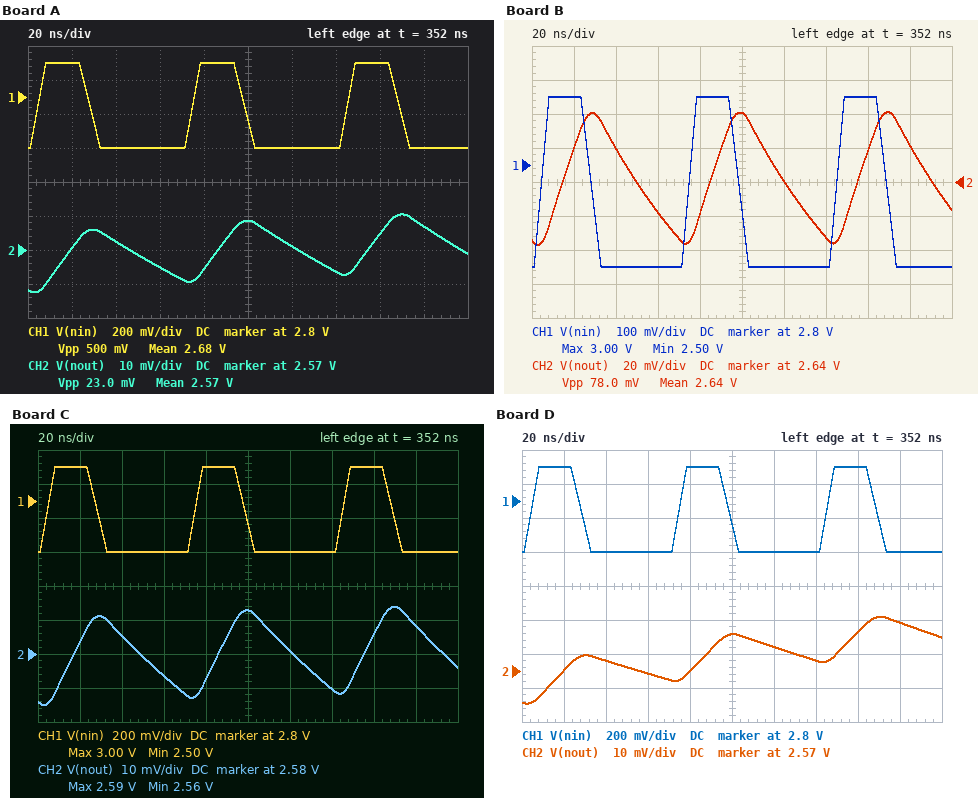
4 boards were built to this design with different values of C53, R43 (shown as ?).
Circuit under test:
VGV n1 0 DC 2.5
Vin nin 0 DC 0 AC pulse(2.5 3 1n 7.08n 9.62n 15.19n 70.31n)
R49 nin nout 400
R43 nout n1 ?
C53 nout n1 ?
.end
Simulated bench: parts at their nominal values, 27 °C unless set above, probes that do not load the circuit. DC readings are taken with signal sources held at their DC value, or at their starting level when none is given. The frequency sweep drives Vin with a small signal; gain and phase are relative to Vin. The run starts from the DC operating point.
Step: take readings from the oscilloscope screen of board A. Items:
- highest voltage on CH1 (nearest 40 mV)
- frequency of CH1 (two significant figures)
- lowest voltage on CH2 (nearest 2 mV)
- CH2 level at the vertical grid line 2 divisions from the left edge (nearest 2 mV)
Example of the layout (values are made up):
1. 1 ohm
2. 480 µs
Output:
1. 3.00 V
2. 14 MHz
3. 2.558 V
4. 2.572 V
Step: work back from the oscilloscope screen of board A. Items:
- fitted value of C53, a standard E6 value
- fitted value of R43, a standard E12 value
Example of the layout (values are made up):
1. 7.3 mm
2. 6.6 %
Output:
1. 1 nF
2. 330 Ω
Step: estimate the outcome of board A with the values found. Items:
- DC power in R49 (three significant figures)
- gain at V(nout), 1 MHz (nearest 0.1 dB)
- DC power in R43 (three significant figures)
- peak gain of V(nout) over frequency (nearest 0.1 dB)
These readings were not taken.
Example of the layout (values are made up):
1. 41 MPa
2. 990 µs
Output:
1. 4.69 mW
2. -10.5 dB
3. 3.87 mW
4. -6.9 dB
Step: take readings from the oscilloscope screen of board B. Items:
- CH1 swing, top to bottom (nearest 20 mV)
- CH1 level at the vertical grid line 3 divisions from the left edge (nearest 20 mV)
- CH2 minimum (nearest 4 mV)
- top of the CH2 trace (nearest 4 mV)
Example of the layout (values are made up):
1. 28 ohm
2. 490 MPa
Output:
1. 500 mV
2. 2.50 V
3. 2.604 V
4. 2.680 V
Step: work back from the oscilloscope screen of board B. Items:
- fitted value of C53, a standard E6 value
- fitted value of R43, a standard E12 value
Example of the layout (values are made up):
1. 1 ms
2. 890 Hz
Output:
1. 220 pF
2. 2.2 kΩ
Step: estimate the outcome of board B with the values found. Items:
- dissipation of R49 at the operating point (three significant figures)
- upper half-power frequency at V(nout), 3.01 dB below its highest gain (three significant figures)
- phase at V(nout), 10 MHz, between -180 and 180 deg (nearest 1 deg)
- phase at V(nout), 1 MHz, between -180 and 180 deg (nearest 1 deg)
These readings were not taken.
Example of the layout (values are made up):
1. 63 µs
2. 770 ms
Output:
1. 370 µW
2. 2.14 MHz
3. -78 deg
4. -25 deg
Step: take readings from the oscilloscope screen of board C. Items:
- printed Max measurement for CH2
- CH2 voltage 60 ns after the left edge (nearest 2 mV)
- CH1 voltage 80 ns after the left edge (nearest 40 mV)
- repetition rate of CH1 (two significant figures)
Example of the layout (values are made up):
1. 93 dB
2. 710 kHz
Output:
1. 2.59 V
2. 2.574 V
3. 3.00 V
4. 14 MHz
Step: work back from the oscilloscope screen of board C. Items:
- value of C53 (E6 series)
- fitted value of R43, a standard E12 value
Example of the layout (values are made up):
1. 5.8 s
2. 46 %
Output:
1. 680 pF
2. 390 Ω
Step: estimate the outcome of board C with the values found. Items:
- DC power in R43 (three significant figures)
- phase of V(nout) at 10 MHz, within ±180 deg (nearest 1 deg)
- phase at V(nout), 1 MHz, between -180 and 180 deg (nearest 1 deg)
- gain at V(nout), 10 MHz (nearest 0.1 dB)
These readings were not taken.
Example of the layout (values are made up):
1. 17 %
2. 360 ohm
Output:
1. 3.91 mW
2. -83 deg
3. -40 deg
4. -24.7 dB
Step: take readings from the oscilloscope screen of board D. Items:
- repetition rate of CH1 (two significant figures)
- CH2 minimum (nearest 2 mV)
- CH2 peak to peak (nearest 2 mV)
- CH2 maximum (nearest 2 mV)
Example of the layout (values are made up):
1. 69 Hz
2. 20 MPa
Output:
1. 14 MHz
2. 2.560 V
3. 26 mV
4. 2.586 V
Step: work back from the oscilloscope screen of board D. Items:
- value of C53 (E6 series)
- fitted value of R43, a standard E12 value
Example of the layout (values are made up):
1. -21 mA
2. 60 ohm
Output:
1. 1.5 nF
2. 680 Ω
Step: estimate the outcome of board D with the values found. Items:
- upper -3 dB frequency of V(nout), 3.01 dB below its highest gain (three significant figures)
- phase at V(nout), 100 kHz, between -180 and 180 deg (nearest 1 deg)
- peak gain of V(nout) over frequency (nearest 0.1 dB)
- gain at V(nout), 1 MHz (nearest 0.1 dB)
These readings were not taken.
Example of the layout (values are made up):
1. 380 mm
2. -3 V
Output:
1. 421 kHz
2. -13 deg
3. -4.0 dB
4. -12.2 dB
